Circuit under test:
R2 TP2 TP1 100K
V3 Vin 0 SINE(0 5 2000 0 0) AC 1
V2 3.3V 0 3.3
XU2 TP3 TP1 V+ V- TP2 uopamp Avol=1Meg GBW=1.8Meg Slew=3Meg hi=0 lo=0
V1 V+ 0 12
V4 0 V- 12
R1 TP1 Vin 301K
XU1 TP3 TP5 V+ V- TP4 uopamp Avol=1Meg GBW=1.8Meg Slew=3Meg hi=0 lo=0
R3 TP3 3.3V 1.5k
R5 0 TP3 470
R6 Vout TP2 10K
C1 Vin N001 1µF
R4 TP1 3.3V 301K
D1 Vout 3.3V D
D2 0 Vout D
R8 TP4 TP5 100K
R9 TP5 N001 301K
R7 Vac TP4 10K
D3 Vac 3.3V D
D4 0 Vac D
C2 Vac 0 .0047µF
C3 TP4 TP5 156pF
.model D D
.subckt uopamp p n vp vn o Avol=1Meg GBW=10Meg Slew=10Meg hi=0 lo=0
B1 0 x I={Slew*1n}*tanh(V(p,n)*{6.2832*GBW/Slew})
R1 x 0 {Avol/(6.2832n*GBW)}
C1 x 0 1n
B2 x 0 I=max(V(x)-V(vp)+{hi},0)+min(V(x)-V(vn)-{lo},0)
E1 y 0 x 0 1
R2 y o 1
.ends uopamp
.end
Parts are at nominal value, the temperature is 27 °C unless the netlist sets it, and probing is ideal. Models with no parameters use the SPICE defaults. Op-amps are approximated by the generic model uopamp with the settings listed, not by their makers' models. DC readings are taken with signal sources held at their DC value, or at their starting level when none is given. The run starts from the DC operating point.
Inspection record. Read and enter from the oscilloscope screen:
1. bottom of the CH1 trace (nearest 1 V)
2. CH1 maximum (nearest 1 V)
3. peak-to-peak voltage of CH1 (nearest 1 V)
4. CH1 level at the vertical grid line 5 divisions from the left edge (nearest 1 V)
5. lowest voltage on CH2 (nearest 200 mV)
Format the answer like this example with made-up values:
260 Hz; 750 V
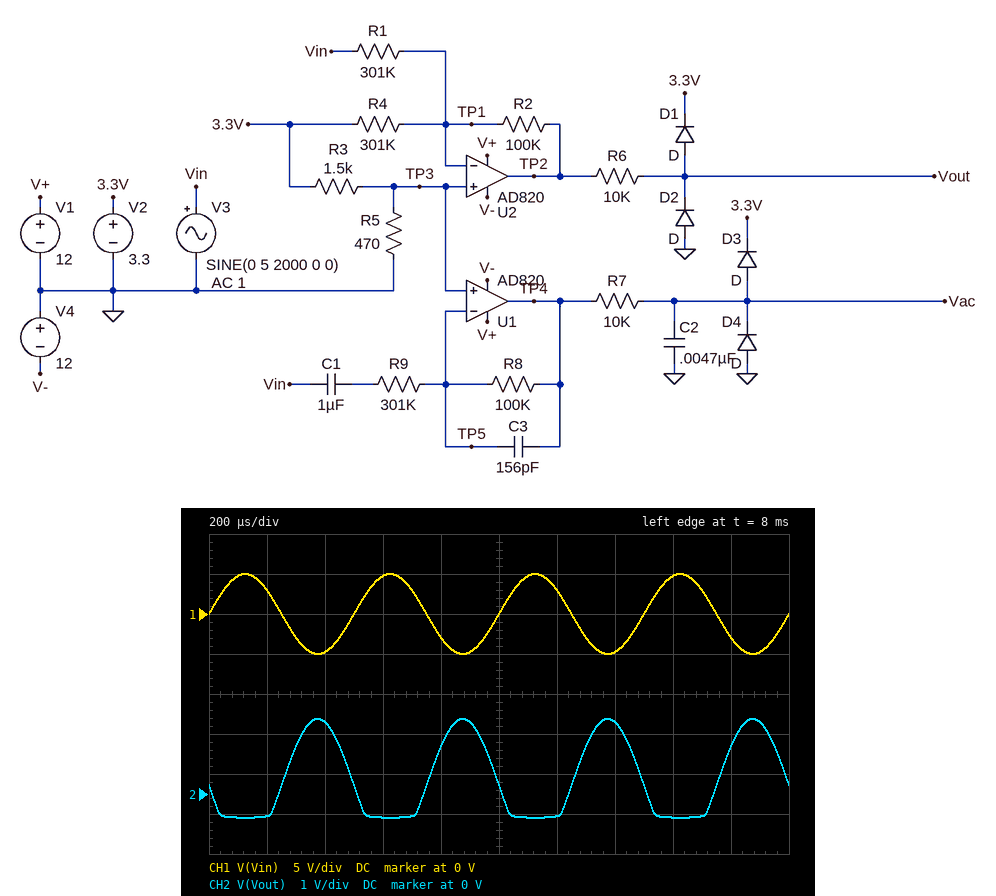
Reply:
-5 V; 5 V; 10 V; 0 V; -600 mV
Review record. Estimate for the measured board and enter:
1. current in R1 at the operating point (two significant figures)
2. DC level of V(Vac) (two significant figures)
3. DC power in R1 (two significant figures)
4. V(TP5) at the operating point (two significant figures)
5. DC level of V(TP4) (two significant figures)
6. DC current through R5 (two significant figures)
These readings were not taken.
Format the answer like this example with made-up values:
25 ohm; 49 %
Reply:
2.6 µA; 790 mV; 2.1 µW; 790 mV; 790 mV; 1.7 mA
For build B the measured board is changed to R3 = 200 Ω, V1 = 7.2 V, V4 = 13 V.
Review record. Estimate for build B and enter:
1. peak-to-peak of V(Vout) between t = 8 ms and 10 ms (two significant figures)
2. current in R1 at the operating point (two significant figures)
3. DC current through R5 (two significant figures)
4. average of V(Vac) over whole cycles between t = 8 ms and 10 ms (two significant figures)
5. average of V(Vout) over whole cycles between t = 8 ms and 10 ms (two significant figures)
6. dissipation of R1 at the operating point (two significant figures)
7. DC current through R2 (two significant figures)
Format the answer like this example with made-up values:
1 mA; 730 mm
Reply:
2.8 V; 7.7 µA; 4.9 mA; 2.3 V; 2.7 V; 18 µW; 4.4 µA
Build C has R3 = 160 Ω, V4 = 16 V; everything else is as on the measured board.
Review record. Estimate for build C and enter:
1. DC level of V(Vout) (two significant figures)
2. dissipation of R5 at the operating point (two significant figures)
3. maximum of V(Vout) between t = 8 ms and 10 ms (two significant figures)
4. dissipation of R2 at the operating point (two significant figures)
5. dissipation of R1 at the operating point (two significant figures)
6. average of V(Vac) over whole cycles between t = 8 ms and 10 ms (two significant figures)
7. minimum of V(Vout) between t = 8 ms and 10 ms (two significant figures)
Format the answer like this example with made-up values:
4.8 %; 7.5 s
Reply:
3.0 V; 13 mW; 3.9 V; 2.9 µW; 20 µW; 2.5 V; 1.3 V
